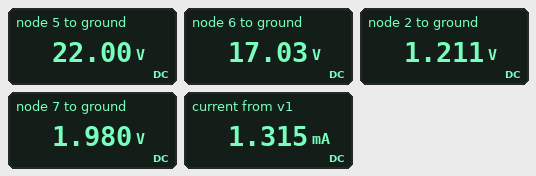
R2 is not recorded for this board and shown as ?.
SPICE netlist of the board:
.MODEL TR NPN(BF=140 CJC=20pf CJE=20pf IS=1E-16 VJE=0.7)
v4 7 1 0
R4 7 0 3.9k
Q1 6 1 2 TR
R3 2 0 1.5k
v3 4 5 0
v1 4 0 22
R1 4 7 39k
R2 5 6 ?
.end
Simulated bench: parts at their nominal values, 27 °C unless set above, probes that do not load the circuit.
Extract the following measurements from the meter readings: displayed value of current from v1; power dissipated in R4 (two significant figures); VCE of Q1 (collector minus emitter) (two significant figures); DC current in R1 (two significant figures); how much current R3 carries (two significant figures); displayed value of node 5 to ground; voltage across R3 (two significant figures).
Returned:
1.315 mA
1.0 mW
16 V
510 µA
810 µA
22.00 V
1.2 V
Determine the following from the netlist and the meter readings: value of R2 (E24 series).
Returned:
6.2 kΩ
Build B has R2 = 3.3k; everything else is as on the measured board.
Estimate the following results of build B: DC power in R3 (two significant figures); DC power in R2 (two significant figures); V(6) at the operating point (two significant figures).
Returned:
980 µW
2.1 mW
19 V
